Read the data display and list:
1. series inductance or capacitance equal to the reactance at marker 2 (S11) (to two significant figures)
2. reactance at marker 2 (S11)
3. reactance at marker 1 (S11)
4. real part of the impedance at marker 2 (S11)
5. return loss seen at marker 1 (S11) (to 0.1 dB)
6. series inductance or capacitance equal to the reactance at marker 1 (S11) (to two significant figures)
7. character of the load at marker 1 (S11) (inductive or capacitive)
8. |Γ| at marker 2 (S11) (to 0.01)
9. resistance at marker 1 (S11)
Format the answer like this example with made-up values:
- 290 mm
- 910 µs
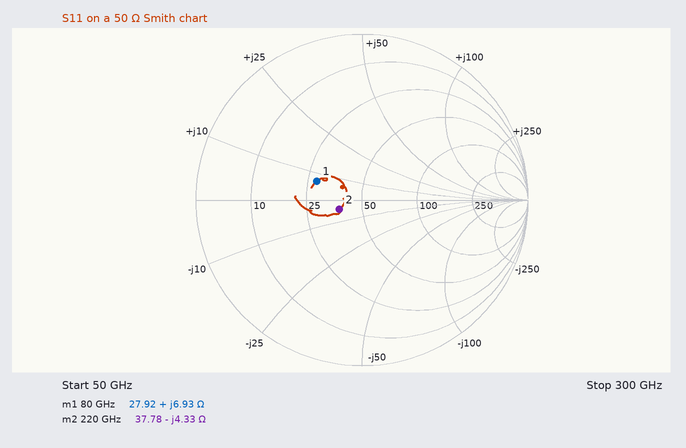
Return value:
- 170 fF
- -4.33 Ω
- +6.93 Ω
- 37.78 Ω
- 10.6 dB
- 14 pH
- inductive
- 0.15
- 27.92 Ω
